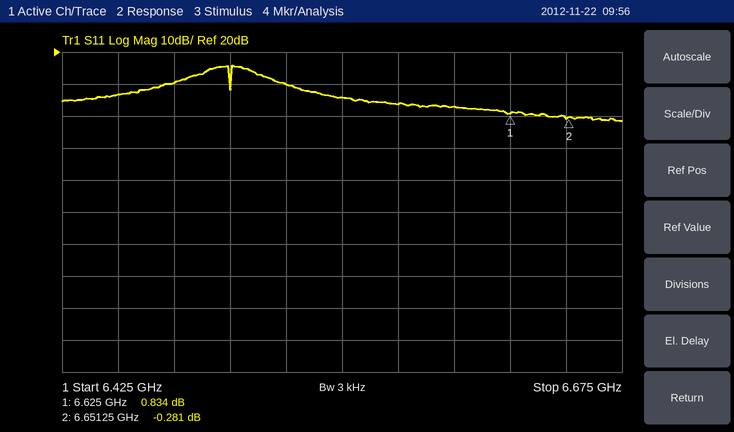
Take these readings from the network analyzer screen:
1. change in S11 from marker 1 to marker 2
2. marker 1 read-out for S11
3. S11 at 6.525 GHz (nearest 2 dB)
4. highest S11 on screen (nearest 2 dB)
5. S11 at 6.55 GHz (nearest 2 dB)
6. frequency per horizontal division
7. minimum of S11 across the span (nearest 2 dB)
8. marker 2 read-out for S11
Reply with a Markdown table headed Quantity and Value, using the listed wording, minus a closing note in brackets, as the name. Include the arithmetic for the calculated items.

| Quantity | Value |
|---|---|
| change in S11 from marker 1 to marker 2 | -0.281 − (0.834) = -1.115 dB |
| marker 1 read-out for S11 | 0.834 dB |
| S11 at 6.525 GHz | 10 dB |
| highest S11 on screen | 16 dB |
| S11 at 6.55 GHz | 6 dB |
| frequency per horizontal division | 25 MHz |
| minimum of S11 across the span | -2 dB |
| marker 2 read-out for S11 | -0.281 dB |
